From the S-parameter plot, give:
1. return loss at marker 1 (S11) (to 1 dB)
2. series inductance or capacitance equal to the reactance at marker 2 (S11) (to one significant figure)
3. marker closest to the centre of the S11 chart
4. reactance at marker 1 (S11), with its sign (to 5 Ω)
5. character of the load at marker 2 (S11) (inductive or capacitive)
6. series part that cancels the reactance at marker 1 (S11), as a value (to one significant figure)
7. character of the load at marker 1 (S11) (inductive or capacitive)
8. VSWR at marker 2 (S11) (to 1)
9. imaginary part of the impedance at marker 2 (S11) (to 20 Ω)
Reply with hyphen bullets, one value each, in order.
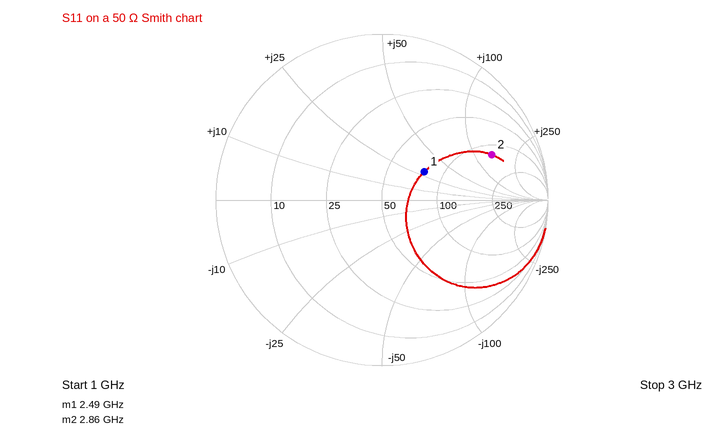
- 10 dB
- 8 nH
- marker 1
- +30 Ω
- inductive
- 2 pF
- inductive
- 6
- +140 Ω
